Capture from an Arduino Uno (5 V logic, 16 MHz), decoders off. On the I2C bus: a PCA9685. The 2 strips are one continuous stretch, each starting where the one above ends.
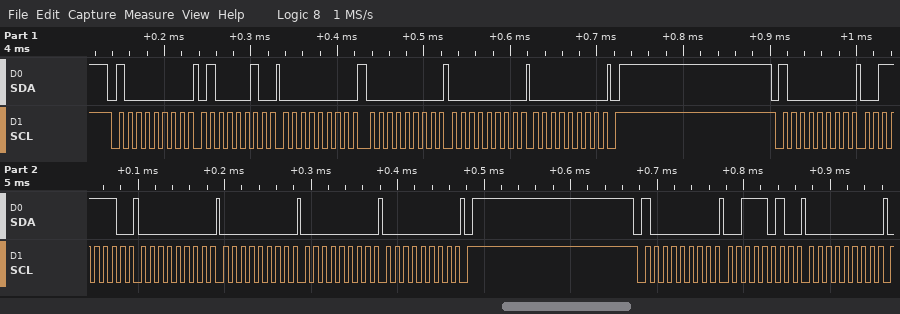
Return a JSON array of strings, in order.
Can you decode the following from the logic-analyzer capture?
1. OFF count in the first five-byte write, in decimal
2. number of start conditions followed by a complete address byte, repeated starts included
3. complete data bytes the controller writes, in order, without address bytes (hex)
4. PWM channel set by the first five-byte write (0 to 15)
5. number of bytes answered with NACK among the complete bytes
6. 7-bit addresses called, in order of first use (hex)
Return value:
["0", "3", "42 00 00 00 00 3E 00 00 00 00 3A 00", "15", "0", "0x40"]
